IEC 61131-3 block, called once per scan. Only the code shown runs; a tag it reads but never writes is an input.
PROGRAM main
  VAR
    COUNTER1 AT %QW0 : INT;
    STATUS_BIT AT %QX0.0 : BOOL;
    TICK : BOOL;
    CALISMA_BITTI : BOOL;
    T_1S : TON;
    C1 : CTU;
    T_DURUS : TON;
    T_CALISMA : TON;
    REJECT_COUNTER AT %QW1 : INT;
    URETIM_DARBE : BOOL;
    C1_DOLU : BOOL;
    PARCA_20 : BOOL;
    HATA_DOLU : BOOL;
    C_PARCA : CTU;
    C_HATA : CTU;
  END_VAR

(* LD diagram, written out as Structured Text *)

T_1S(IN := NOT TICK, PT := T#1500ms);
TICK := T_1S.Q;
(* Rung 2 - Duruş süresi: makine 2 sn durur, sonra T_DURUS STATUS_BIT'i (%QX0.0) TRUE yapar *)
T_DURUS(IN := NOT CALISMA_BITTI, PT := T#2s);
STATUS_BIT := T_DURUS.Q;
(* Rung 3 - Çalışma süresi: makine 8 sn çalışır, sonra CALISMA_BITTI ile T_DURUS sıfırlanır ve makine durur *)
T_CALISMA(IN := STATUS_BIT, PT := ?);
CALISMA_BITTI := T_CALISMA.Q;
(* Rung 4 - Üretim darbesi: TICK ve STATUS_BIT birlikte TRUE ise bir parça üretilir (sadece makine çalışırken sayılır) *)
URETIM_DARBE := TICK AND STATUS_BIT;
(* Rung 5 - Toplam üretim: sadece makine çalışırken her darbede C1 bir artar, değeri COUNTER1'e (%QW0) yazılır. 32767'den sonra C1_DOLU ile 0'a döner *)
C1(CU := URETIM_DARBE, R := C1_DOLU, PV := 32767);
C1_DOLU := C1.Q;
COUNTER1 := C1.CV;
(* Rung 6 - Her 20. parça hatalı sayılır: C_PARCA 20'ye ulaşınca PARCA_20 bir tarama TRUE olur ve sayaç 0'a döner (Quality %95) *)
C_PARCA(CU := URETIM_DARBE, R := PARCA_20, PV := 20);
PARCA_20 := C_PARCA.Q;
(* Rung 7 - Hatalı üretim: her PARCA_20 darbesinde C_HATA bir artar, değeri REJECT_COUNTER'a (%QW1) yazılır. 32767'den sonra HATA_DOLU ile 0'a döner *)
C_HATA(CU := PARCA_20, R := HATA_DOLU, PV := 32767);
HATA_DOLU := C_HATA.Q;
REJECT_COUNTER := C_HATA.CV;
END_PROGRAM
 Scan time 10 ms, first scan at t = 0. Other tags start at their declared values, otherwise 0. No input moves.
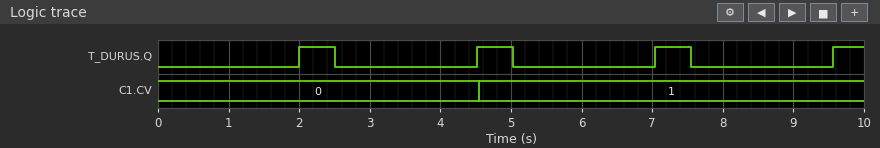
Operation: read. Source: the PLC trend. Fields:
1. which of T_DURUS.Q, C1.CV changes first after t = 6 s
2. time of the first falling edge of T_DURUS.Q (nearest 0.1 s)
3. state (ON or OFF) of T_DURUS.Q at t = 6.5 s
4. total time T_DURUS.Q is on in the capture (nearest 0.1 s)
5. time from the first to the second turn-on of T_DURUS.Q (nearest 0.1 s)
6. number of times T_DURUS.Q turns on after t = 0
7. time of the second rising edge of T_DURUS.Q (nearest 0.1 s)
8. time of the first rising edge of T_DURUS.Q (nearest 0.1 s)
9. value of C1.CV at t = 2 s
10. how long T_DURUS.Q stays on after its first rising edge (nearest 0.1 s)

T_DURUS.Q
2.5 s
OFF
2.0 s
2.5 s
4
4.5 s
2.0 s
0
0.5 s
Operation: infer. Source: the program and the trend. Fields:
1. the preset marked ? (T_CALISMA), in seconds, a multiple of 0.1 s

0.5 s
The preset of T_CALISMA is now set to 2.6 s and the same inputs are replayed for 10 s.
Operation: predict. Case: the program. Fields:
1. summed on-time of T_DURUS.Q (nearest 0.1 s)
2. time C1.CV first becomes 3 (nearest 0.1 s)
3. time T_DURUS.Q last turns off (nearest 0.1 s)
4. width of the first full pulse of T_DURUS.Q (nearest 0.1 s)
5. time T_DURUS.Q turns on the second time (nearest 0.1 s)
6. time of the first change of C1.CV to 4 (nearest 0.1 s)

5.2 s
7.6 s
9.2 s
2.6 s
6.6 s
9.1 s
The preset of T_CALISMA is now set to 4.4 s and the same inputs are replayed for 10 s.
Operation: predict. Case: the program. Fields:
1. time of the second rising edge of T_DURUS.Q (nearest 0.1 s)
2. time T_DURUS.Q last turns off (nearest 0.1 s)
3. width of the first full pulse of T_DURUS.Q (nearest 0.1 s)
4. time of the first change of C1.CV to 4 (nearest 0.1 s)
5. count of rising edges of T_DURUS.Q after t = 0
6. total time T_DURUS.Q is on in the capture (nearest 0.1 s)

8.4 s
6.4 s
4.4 s
9.1 s
2
6.0 s
